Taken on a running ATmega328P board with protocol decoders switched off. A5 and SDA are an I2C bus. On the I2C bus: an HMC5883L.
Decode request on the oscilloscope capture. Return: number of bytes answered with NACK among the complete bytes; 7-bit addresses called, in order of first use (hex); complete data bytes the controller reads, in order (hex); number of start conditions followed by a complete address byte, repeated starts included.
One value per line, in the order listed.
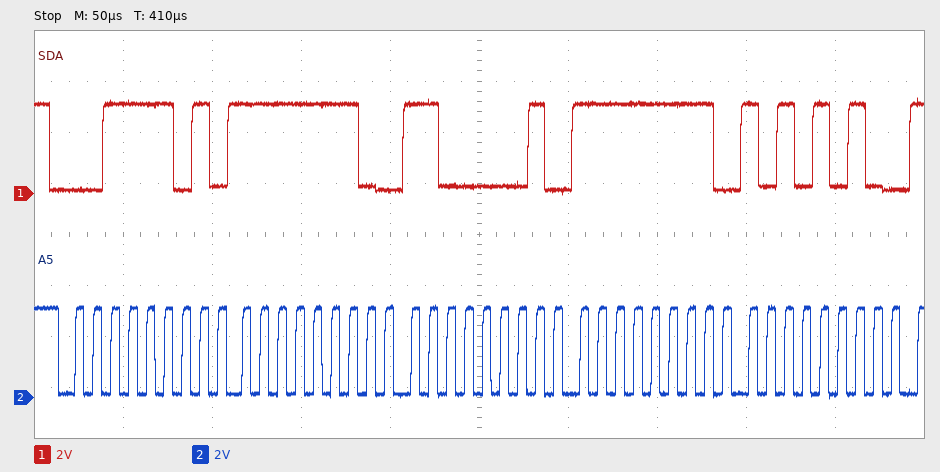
0
0x1E
FE C1 FF AA
1
